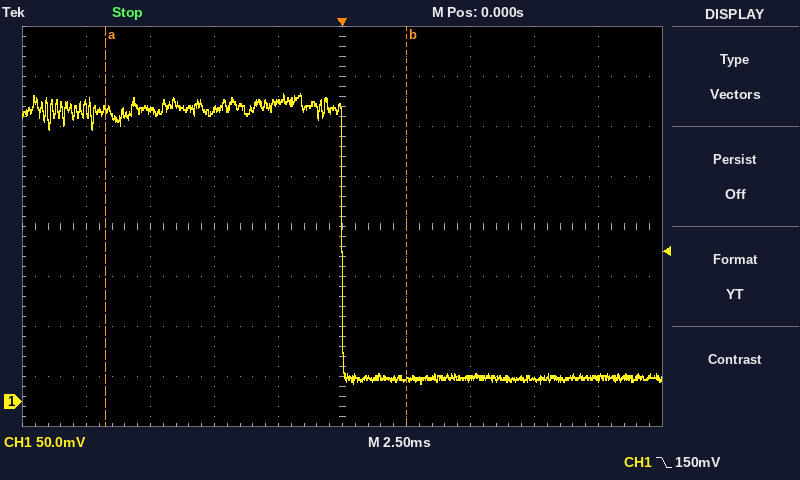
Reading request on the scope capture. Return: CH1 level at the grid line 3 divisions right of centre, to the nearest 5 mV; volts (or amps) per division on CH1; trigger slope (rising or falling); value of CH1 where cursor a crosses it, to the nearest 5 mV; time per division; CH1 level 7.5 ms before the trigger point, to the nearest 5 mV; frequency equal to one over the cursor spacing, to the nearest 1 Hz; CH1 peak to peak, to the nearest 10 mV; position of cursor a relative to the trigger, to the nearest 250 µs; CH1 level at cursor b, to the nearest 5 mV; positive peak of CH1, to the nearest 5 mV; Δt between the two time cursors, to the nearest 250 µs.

20 mV
50 mV
falling
290 mV
2.5 ms
290 mV
85 Hz
290 mV
-9.25 ms
20 mV
310 mV
11.75 ms
